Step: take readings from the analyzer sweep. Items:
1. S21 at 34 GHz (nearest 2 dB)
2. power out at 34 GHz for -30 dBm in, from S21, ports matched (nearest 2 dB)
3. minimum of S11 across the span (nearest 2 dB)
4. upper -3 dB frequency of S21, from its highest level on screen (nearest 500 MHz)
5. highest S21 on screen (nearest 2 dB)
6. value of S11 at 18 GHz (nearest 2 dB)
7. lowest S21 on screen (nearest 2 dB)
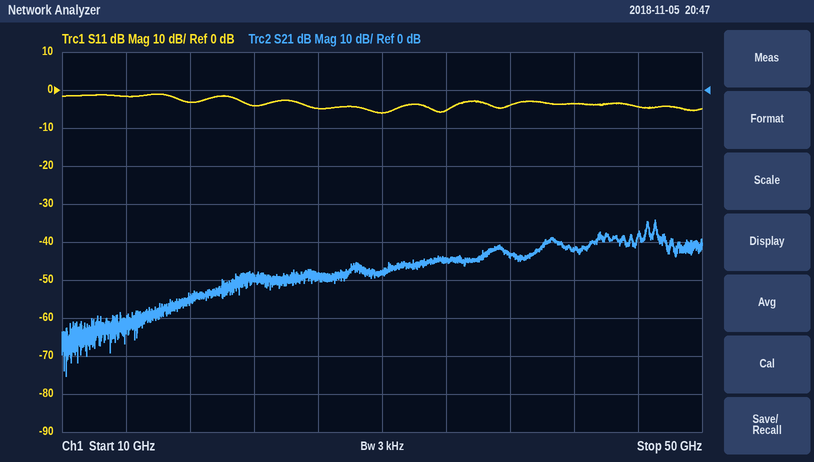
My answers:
-44 dB
-74 dBm
-6 dB
47.0 GHz
-34 dB
-4 dB
-76 dB
